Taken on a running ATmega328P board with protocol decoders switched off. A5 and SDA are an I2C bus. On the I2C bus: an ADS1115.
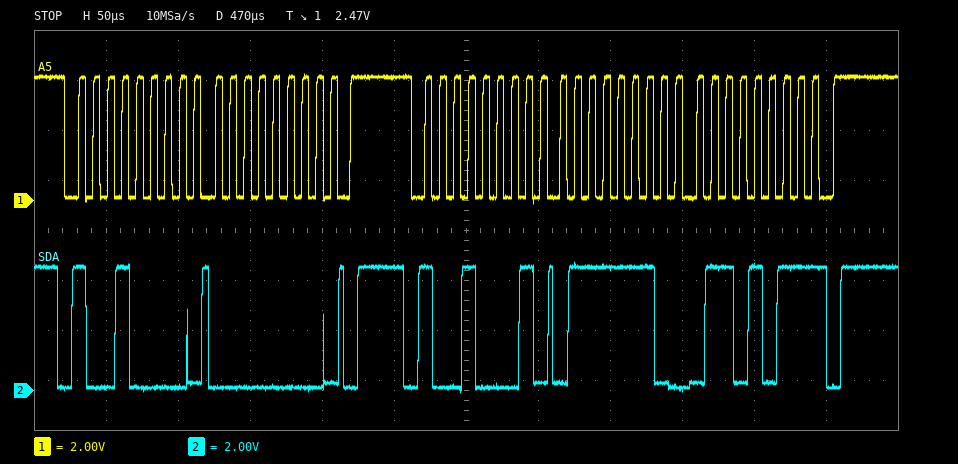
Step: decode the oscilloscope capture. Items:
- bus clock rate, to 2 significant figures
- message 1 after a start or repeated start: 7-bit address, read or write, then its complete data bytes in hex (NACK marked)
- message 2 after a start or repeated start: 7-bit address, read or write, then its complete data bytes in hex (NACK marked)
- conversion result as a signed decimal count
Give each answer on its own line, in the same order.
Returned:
100 kHz
0x48 write: 00
0x48 read: 7E 6B NACK
32363
